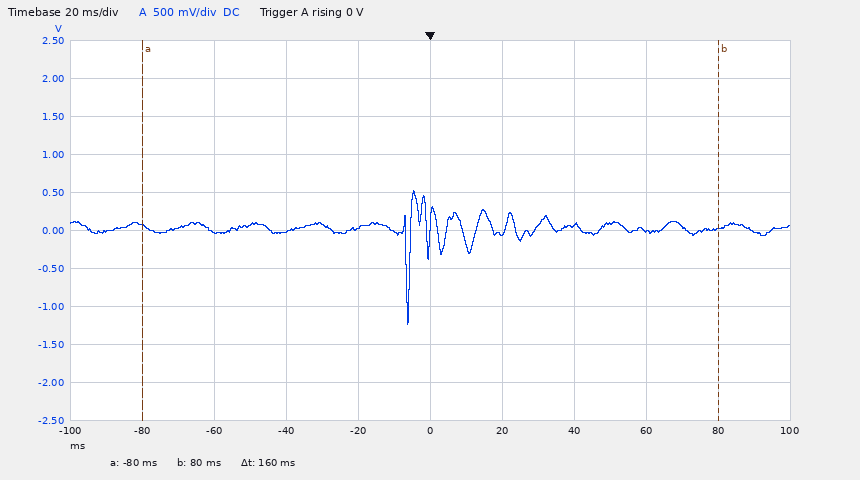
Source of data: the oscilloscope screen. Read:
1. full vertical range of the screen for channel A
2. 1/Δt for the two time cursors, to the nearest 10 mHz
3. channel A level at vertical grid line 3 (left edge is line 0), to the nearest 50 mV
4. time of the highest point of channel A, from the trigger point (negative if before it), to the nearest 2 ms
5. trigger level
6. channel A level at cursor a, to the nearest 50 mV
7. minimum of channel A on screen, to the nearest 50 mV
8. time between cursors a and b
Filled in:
5 V
6.25 Hz
0 mV
-4 ms
0 V
50 mV
-1.25 V
160 ms
